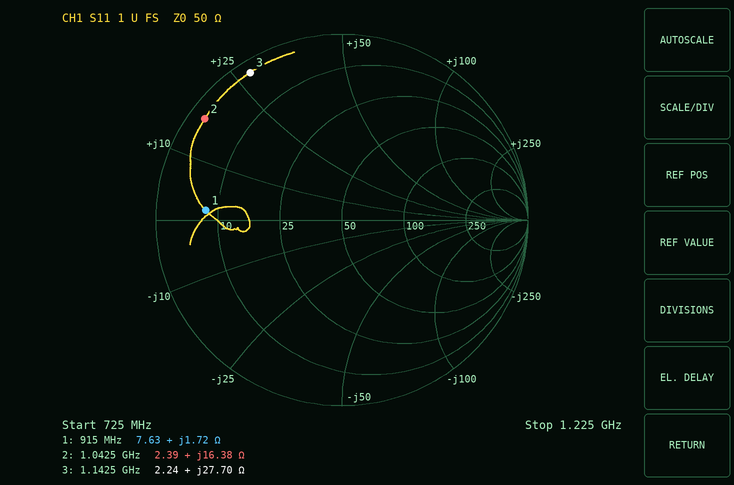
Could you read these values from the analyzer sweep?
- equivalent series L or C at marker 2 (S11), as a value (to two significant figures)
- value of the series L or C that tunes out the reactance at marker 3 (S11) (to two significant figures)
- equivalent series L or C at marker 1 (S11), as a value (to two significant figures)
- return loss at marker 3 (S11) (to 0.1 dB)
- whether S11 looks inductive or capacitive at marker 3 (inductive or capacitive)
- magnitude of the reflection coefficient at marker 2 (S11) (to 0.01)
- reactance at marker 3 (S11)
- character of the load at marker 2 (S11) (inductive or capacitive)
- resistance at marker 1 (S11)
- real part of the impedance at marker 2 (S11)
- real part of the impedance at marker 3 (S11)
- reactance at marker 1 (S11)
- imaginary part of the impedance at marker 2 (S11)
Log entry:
2.5 nH
5.0 pF
300 pH
0.6 dB
inductive
0.92
+27.70 Ω
inductive
7.63 Ω
2.39 Ω
2.24 Ω
+1.72 Ω
+16.38 Ω
